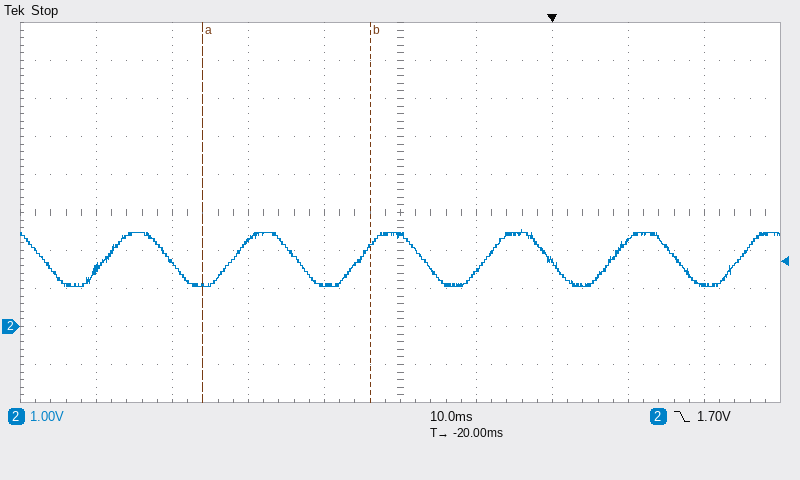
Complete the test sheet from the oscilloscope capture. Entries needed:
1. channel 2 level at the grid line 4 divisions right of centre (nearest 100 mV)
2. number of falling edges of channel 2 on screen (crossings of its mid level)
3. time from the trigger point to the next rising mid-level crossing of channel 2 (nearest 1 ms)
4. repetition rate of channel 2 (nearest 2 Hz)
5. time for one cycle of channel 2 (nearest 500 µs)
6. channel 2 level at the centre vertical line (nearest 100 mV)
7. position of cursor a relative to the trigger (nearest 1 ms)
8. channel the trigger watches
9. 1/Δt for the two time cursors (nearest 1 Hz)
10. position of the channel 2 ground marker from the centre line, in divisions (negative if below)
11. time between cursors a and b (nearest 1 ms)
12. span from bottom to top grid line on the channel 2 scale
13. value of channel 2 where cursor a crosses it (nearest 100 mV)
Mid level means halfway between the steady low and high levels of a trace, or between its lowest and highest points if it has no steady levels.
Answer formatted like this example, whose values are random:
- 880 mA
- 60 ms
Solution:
- 1.1 V
- 6
- 8 ms
- 60 Hz
- 16.5 ms
- 2.4 V
- -46 ms
- channel 2
- 45 Hz
- -3.0 div
- 22 ms
- 10 V
- 1.1 V
